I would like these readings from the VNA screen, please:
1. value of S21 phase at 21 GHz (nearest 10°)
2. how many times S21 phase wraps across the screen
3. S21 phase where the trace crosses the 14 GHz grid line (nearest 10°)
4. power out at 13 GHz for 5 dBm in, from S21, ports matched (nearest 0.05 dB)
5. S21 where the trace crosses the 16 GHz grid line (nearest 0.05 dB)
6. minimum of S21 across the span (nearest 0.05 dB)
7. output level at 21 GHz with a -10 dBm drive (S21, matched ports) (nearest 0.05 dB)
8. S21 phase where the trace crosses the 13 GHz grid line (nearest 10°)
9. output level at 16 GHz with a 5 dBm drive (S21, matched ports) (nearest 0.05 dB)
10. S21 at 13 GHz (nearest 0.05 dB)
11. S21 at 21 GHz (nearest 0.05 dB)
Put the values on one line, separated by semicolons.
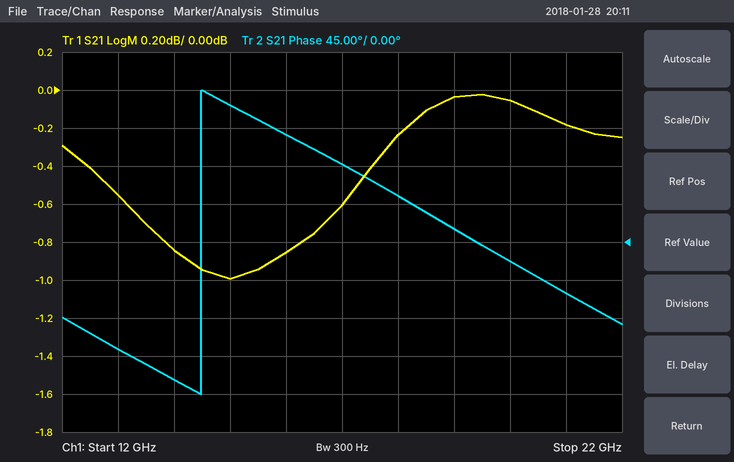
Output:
-60°; 1; -160°; 4.45 dBm; -0.85 dB; -1.00 dB; -10.20 dBm; -130°; 4.15 dBm; -0.55 dB; -0.20 dB
